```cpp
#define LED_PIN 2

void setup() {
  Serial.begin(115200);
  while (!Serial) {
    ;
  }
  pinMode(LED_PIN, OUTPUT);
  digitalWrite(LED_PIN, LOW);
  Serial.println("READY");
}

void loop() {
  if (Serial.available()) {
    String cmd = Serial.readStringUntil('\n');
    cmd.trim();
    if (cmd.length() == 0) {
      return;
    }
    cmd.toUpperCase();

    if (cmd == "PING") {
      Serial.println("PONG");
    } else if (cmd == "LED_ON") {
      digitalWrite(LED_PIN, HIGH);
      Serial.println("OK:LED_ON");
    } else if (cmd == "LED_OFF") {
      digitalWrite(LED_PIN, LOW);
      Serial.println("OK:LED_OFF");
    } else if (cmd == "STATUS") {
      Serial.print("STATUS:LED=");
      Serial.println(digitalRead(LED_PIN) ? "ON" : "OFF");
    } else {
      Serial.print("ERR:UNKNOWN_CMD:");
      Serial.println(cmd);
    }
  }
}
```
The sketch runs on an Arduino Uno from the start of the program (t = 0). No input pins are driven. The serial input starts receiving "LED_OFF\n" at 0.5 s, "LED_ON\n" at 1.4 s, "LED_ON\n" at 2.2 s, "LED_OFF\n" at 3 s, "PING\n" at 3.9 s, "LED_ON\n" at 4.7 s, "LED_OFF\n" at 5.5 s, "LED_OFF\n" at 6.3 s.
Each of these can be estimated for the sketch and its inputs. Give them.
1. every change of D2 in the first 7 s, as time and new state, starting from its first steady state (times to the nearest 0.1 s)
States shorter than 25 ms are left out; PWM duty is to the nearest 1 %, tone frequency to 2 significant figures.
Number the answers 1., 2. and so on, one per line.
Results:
1. 0 s low; 1.4 s high; 3 s low; 4.7 s high; 5.5 s low
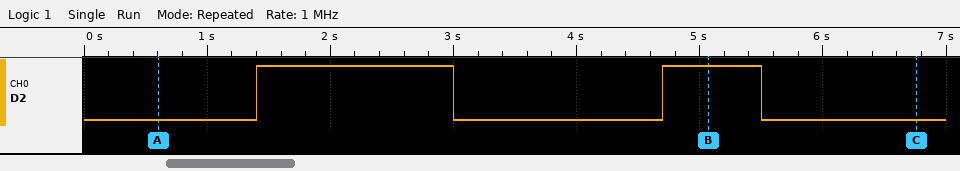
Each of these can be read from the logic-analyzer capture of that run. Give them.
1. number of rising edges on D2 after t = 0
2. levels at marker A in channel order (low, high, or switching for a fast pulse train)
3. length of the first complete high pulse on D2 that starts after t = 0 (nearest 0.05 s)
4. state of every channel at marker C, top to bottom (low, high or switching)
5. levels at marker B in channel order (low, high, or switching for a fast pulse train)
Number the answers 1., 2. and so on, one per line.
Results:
1. 2
2. D2 low
3. 1.60 s
4. D2 low
5. D2 high
